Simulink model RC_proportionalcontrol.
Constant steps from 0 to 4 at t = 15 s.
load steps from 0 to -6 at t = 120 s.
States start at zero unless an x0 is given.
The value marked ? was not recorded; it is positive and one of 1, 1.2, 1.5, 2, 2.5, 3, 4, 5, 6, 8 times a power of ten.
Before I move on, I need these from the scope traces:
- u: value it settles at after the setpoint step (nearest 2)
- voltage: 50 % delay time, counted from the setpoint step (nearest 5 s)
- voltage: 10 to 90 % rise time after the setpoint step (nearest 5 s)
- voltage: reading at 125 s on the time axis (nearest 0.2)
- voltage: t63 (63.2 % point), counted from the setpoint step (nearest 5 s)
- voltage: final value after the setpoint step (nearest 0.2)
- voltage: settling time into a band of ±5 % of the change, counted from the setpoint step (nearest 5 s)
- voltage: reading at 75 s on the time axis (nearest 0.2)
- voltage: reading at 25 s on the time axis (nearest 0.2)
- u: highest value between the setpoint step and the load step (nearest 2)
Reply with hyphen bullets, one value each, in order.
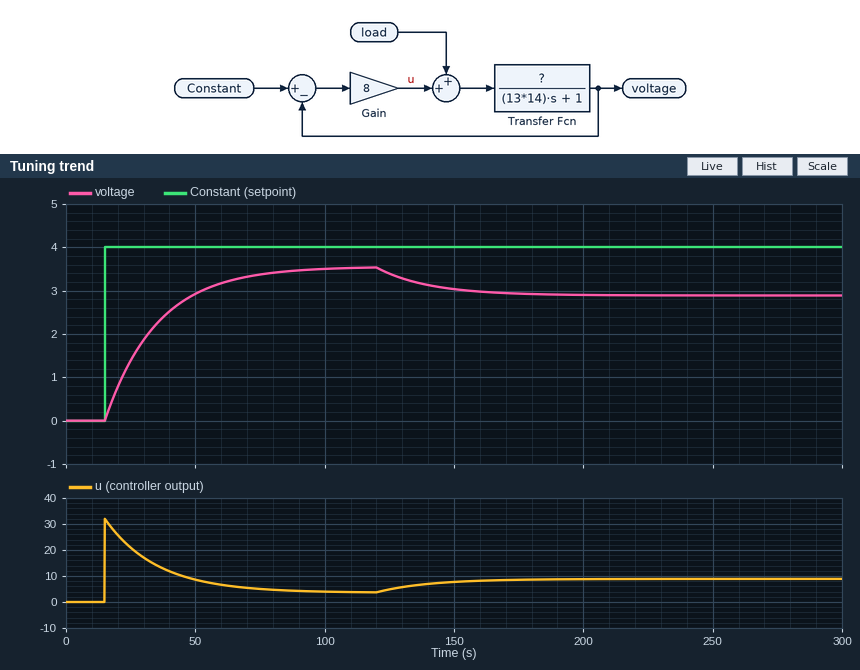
- 4
- 15 s
- 45 s
- 3.4
- 20 s
- 3.6
- 60 s
- 3.4
- 1.4
- 32
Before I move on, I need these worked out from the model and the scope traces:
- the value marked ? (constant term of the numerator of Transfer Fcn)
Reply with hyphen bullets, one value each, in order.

- 1
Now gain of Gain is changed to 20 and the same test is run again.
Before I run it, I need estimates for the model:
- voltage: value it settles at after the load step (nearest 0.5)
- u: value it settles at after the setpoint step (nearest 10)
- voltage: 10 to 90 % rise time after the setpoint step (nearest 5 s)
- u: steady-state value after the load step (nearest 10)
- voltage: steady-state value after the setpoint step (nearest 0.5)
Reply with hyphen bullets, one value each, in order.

- 3.5
- 0
- 20 s
- 10
- 4.0
